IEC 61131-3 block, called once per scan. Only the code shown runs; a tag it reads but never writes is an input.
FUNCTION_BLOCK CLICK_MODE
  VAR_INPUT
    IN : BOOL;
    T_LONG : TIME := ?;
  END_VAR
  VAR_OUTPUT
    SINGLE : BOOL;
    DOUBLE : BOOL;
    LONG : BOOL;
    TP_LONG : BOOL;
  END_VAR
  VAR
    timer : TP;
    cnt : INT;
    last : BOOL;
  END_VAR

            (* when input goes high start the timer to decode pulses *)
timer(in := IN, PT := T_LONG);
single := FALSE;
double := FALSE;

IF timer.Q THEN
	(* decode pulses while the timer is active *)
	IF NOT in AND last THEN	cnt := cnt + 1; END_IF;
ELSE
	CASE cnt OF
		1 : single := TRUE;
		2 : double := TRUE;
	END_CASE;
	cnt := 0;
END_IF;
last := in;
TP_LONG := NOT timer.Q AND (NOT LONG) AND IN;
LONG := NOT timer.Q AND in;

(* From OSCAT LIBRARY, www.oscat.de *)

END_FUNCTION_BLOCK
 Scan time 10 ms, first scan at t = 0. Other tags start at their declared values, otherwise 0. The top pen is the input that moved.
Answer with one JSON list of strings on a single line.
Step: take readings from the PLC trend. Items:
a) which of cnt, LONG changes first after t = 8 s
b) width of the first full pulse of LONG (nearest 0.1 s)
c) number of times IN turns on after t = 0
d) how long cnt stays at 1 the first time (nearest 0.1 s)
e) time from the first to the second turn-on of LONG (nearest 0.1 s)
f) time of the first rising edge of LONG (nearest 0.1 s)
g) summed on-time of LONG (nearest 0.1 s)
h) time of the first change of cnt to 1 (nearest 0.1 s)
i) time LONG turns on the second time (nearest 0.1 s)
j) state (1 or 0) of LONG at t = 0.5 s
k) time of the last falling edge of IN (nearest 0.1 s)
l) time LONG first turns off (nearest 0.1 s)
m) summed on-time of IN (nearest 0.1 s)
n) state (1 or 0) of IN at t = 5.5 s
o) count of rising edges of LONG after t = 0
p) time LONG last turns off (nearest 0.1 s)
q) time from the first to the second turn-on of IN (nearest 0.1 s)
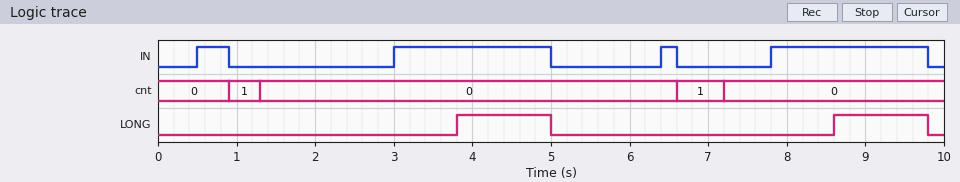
["LONG", "1.2 s", "4", "0.4 s", "4.8 s", "3.8 s", "2.4 s", "0.9 s", "8.6 s", "0", "9.8 s", "5.0 s", "4.6 s", "0", "2", "9.8 s", "2.5 s"]
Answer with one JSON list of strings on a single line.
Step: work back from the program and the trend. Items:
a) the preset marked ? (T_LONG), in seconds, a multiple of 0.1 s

["0.8 s"]
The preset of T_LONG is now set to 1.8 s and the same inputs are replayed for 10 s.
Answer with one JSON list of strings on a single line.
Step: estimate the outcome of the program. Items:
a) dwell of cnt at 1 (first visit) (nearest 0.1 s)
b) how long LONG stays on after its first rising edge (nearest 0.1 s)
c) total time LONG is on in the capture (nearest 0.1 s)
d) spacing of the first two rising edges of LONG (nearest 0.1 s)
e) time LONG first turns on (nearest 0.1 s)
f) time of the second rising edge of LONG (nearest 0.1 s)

["1.4 s", "0.2 s", "1.8 s", "3.4 s", "4.8 s", "8.2 s"]
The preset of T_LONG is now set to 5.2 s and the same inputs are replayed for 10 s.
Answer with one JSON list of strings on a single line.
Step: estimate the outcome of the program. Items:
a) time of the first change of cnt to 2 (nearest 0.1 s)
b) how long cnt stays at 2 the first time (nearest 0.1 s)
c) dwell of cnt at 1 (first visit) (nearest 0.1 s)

["5.0 s", "0.7 s", "4.1 s"]
